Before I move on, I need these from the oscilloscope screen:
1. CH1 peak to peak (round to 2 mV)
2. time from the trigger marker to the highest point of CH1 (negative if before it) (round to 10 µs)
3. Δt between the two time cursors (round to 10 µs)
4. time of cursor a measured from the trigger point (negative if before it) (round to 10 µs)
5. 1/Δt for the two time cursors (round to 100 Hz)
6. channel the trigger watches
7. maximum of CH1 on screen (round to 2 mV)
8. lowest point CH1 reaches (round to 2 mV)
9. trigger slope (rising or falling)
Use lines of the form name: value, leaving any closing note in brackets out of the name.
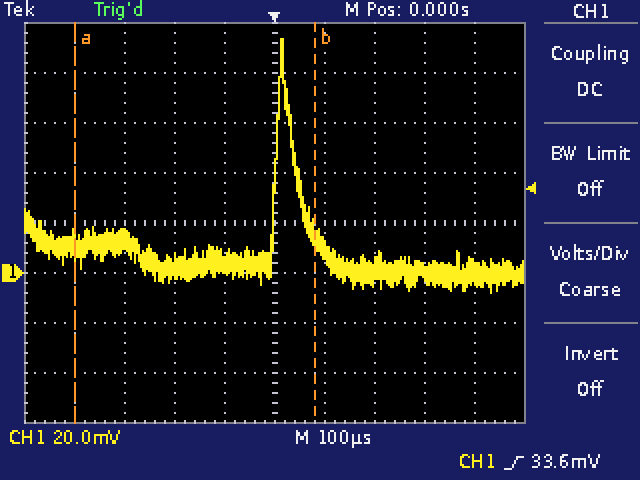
CH1 peak to peak: 102 mV
time from the trigger marker to the highest point of CH1 (negative if before it): +20 µs
Δt between the two time cursors: 480 µs
time of cursor a measured from the trigger point (negative if before it): -400 µs
1/Δt for the two time cursors: 2.1 kHz
channel the trigger watches: CH1
maximum of CH1 on screen: 94 mV
lowest point CH1 reaches: -8 mV
trigger slope: rising
